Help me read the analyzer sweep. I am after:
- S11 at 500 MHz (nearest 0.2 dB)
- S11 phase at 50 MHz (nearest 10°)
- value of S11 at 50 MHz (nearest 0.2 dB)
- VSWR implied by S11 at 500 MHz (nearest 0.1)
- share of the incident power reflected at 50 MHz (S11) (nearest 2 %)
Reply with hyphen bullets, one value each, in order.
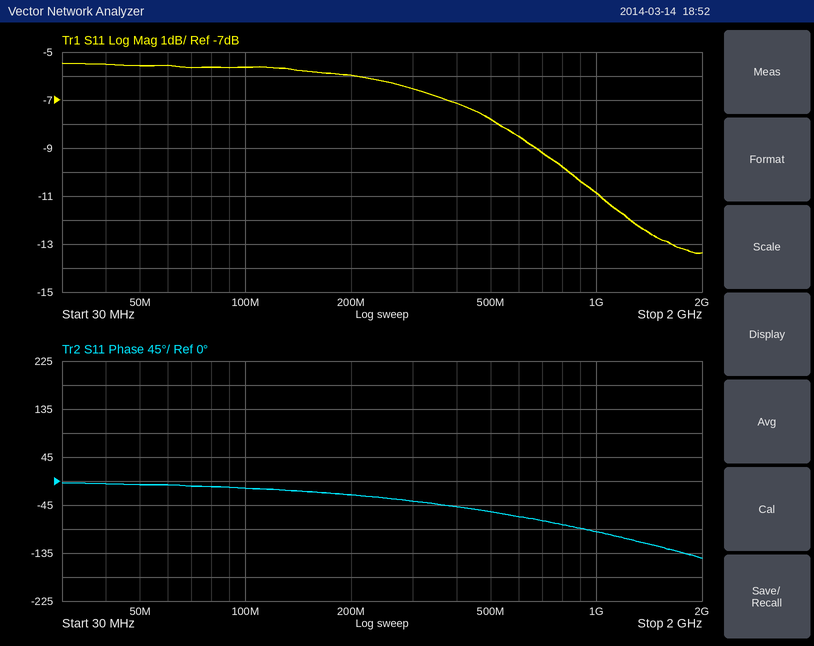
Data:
- -7.8 dB
- -10°
- -5.6 dB
- 2.4
- 28 %
